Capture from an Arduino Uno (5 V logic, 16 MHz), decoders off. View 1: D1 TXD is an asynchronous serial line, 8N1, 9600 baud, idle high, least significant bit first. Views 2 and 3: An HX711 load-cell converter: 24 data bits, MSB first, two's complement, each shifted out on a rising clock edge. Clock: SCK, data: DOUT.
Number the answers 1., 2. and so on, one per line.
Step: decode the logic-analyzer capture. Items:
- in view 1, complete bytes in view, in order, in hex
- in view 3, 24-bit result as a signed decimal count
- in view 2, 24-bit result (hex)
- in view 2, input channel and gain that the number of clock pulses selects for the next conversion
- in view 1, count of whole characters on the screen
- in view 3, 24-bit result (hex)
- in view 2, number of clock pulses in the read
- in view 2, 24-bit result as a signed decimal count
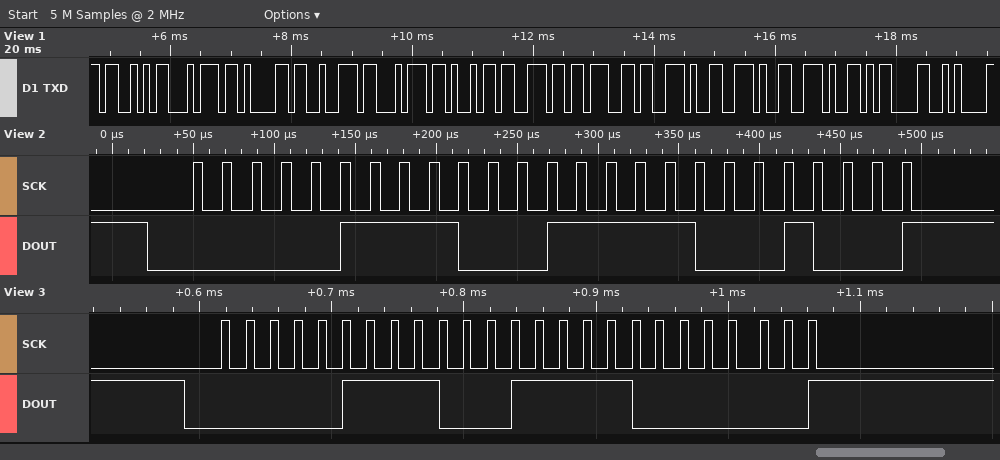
1. 0x53 0x74 0x61 0x72 0x74 0x69 0x6E 0x67 0x2E 0x2E 0x2E 0x0D 0x0A
2. 495488
3. 0x078F88
4. channel A, gain 128
5. 13
6. 0x078F80
7. 25
8. 495496
